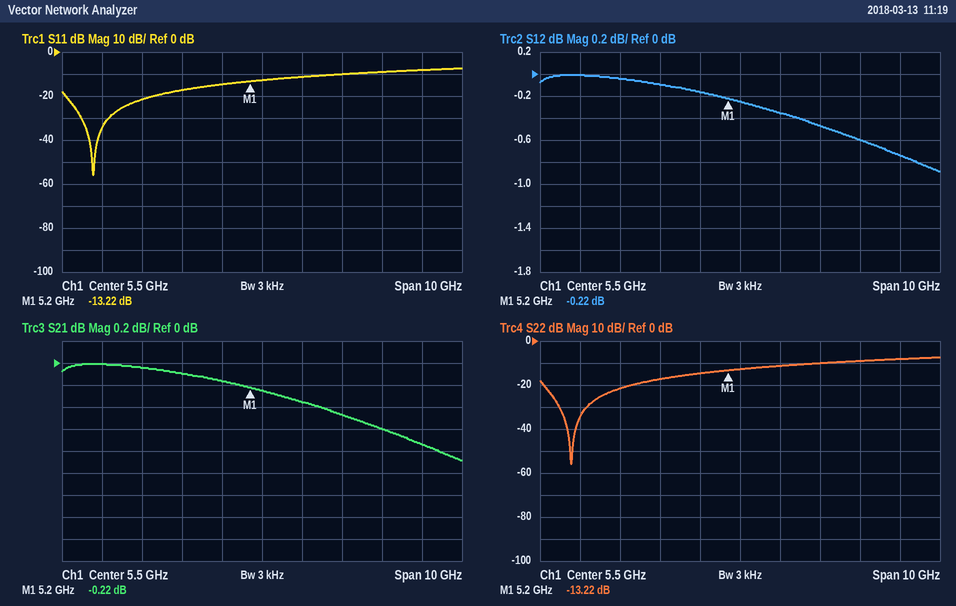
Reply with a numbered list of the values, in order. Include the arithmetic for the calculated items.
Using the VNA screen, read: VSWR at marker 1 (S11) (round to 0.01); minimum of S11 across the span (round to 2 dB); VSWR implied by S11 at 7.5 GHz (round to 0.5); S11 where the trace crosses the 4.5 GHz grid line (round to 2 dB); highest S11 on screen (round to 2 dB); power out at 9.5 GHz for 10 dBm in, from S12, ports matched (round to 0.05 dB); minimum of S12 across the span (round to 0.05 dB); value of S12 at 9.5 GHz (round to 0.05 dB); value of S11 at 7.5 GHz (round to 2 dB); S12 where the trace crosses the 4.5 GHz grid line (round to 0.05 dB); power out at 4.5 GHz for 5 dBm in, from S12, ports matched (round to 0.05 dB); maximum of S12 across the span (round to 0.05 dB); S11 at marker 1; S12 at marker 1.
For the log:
1. (1 + 0.2183)/(1 − 0.2183) ≈ 1.56
2. -56 dB
3. |Γ| = 10^(-10/20) = 0.3162; VSWR = (1 + 0.3162)/(1 − 0.3162) ≈ 1.92, so 2.0 to the nearest 0.5
4. -14 dB
5. -8 dB
6. 10 dBm + (-0.75 dB) = 9.25 dBm
7. -0.90 dB
8. -0.75 dB
9. -10 dB
10. -0.15 dB
11. 5 dBm + (-0.15 dB) = 4.85 dBm
12. 0.00 dB
13. -13.22 dB
14. -0.22 dB
